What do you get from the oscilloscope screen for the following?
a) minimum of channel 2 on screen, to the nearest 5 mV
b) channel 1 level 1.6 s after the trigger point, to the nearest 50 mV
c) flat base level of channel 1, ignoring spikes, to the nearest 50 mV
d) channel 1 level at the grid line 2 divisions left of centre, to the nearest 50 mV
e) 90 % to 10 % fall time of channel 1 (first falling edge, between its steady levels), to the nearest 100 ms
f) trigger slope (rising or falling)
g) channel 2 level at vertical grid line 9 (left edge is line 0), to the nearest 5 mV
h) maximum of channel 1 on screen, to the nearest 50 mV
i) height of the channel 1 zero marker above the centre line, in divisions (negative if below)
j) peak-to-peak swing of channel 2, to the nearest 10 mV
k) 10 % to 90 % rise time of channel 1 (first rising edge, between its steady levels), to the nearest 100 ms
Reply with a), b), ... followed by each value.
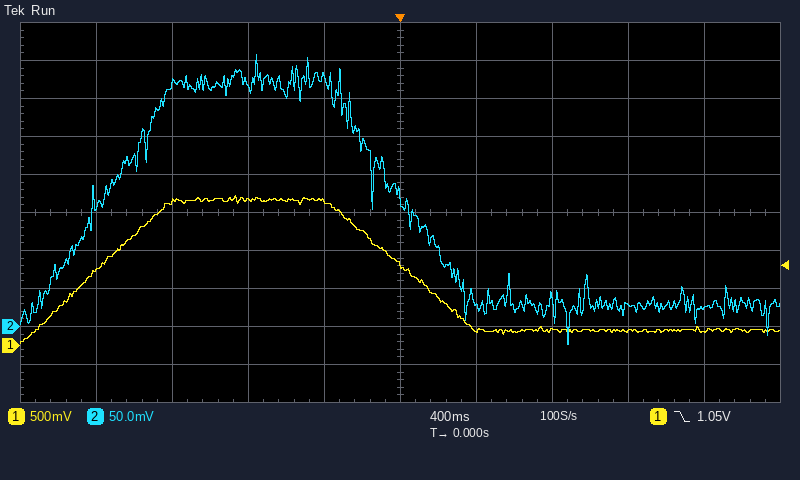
a) -25 mV
b) 200 mV
c) 200 mV
d) 1.90 V
e) 600 ms
f) falling
g) 25 mV
h) 1.95 V
i) -3.5 div
j) 380 mV
k) 600 ms
